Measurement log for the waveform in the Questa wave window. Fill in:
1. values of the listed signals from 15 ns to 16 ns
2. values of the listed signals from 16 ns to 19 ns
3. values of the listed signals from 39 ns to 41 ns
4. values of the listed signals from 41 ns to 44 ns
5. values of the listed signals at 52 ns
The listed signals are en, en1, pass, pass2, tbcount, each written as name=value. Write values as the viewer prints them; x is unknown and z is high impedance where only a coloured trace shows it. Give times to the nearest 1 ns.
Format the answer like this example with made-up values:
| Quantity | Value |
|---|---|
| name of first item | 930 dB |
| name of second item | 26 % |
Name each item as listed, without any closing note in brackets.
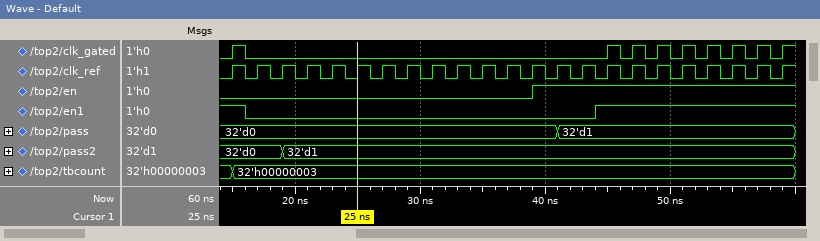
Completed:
| Quantity | Value |
|---|---|
| values of the listed signals from 15 ns to 16 ns | en=0, en1=1, pass=32'd0, pass2=32'd0, tbcount=32'h00000003 |
| values of the listed signals from 16 ns to 19 ns | en=0, en1=0, pass=32'd0, pass2=32'd0, tbcount=32'h00000003 |
| values of the listed signals from 39 ns to 41 ns | en=1, en1=0, pass=32'd0, pass2=32'd1, tbcount=32'h00000003 |
| values of the listed signals from 41 ns to 44 ns | en=1, en1=0, pass=32'd1, pass2=32'd1, tbcount=32'h00000003 |
| values of the listed signals at 52 ns | en=1, en1=1, pass=32'd1, pass2=32'd1, tbcount=32'h00000003 |
